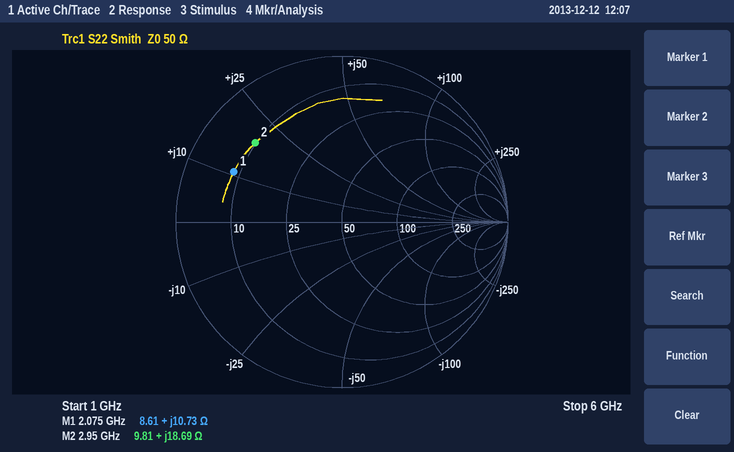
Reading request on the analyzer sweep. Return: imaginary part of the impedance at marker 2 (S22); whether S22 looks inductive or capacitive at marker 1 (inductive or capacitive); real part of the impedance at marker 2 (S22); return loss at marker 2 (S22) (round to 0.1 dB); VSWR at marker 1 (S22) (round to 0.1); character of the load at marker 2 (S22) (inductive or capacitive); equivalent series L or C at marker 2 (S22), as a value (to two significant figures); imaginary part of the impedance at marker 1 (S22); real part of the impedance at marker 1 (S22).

+18.69 Ω
inductive
9.81 Ω
3.0 dB
6.1
inductive
1.0 nH
+10.73 Ω
8.61 Ω
